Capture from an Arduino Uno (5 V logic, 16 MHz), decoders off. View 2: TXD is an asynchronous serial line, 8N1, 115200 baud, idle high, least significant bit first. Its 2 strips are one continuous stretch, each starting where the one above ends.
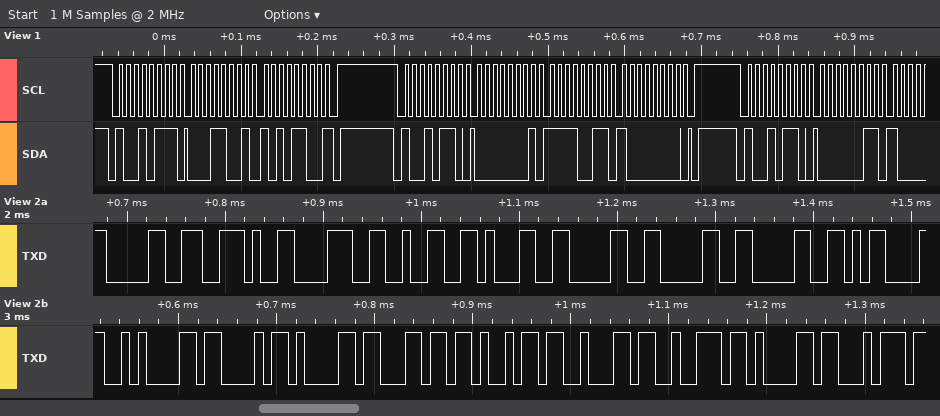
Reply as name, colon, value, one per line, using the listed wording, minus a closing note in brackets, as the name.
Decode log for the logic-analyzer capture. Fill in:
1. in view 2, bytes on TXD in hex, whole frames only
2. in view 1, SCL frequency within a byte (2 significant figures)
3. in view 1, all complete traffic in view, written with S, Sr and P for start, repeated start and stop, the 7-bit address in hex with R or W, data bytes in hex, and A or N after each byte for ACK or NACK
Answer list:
in view 2, bytes on TXD in hex, whole frames only: 30 2E 38 32 31 30 30 30 0D 0A 43 61 6C 69 62 72 61 74
in view 1, SCL frequency within a byte: 100 kHz
in view 1, all complete traffic in view, written with S, Sr and P for start, repeated start and stop, the 7-bit address in hex with R or W, data bytes in hex, and A or N after each byte for ACK or NACK: S 4BR A 19 A AC N P S 4BW A 01 A F3 A 80 A P S 4BW A 03 A
